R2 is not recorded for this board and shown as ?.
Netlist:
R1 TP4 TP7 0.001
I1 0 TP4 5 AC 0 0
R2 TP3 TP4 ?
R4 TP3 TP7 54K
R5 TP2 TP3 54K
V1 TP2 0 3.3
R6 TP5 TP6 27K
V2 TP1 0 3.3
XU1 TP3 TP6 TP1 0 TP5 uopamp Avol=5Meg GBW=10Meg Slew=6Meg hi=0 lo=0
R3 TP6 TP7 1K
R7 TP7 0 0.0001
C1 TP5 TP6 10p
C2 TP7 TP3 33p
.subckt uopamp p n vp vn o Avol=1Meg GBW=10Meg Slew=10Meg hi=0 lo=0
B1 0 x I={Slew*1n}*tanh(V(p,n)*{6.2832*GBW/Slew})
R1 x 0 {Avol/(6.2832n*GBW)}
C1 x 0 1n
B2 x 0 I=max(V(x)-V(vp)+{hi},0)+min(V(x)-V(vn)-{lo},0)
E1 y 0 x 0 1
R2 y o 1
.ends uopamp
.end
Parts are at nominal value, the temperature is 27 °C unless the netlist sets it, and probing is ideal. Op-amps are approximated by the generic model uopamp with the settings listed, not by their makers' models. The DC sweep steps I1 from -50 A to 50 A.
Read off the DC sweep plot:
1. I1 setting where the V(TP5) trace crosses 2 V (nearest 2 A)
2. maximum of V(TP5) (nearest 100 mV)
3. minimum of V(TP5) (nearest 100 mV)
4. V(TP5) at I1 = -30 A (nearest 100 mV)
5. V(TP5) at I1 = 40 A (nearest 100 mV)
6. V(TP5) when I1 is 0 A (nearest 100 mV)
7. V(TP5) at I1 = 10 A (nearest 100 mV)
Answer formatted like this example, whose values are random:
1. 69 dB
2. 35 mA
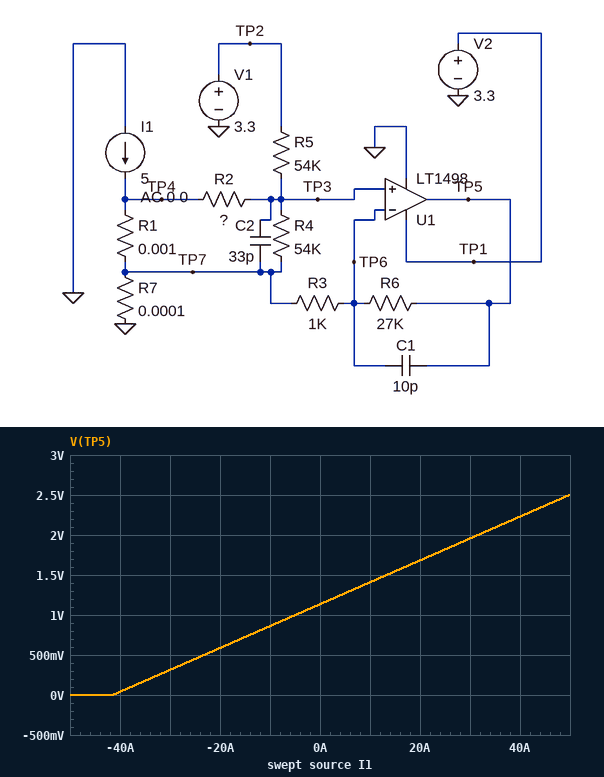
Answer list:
1. 32 A
2. 2.5 V
3. 0 V
4. 300 mV
5. 2.2 V
6. 1.1 V
7. 1.4 V
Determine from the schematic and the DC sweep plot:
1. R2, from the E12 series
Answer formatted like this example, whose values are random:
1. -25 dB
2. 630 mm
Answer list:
1. 680 Ω
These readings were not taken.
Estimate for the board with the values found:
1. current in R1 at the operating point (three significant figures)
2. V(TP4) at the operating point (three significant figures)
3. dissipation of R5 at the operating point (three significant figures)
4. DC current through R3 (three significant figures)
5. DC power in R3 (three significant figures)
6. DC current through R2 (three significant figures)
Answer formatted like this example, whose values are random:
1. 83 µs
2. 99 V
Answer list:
1. 5.00 A
2. 5.50 mV
3. 196 µW
4. 45.4 µA
5. 2.06 µW
6. 59.4 µA
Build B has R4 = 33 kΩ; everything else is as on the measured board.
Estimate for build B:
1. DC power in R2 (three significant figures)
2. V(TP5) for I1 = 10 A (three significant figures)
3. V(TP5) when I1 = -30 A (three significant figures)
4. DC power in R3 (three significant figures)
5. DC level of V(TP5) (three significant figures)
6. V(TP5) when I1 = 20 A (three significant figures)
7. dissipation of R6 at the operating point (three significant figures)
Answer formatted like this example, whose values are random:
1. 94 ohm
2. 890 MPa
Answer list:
1. 2.36 µW
2. 1.40 V
3. 311 mV
4. 2.03 µW
5. 1.26 V
6. 1.67 V
7. 54.8 µW
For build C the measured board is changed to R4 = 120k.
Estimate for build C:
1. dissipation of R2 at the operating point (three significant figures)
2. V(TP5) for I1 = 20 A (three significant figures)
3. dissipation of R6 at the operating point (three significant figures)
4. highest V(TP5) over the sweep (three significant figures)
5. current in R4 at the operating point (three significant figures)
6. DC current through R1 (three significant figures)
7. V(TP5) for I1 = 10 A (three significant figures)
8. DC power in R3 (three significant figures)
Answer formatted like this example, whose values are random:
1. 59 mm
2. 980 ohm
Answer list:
1. 2.44 µW
2. 1.69 V
3. 56.4 µW
4. 2.52 V
5. 381 nA
6. 5.00 A
7. 1.42 V
8. 2.09 µW
